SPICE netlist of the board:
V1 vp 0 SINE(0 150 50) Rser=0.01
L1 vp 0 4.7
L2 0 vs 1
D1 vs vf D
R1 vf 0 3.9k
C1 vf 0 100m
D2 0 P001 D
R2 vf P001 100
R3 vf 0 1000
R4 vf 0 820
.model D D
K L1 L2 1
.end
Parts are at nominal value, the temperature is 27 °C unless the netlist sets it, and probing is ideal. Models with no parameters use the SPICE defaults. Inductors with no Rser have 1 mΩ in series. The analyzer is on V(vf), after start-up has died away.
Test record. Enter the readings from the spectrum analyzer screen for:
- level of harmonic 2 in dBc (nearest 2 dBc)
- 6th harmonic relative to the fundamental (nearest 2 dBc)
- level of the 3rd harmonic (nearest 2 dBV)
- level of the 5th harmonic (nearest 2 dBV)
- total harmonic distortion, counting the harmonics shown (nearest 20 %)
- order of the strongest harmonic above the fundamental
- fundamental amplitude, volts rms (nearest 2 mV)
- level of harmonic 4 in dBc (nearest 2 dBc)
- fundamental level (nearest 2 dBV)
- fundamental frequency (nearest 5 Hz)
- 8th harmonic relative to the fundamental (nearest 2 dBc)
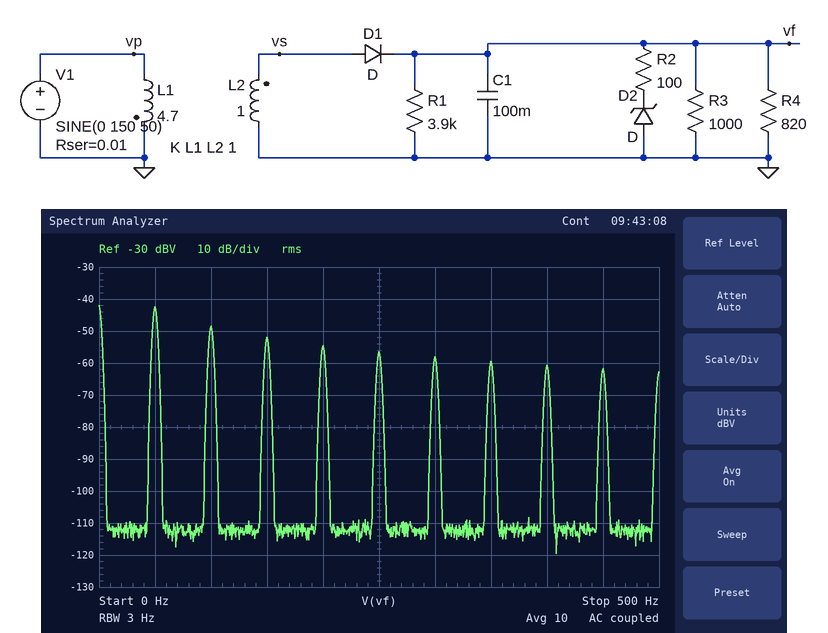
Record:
-6 dBc
-16 dBc
-52 dBV
-56 dBV
80 %
2
8 mV
-12 dBc
-42 dBV
50 Hz
-18 dBc
